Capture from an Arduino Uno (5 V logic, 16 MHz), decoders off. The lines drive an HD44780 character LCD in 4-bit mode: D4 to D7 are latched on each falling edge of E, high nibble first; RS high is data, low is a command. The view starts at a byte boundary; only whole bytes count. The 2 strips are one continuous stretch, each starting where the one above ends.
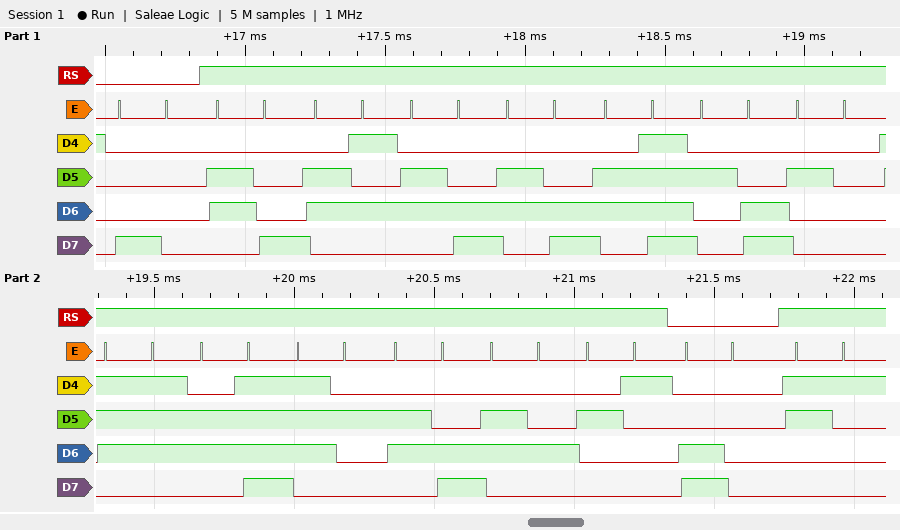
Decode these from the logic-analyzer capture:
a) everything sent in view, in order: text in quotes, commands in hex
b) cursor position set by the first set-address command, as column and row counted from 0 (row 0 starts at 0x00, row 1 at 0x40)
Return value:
0x80 "hello, world!" 0xC0 "1"
column 0, row 0
